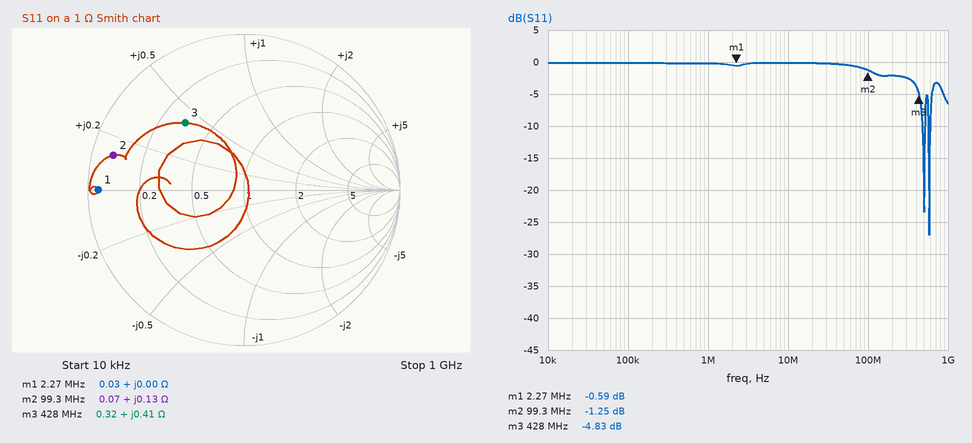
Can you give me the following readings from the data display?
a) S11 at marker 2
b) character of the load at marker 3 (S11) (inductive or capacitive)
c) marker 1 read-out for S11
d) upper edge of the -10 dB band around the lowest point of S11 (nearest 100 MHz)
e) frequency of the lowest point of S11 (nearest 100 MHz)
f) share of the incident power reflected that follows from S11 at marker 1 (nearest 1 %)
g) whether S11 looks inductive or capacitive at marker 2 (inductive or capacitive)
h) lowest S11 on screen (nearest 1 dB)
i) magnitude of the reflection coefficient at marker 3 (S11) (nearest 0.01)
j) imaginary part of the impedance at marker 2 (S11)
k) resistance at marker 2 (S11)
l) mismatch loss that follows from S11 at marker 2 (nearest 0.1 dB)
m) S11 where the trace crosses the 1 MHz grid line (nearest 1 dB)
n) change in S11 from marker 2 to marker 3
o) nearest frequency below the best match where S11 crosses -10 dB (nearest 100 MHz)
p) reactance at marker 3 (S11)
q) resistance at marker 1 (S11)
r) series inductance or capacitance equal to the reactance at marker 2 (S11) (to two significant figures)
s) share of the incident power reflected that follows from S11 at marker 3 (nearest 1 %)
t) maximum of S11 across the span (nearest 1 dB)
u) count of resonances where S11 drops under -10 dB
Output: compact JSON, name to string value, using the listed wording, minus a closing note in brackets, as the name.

{"S11 at marker 2": "-1.25 dB", "character of the load at marker 3 (S11)": "inductive", "marker 1 read-out for S11": "-0.59 dB", "upper edge of the -10 dB band around the lowest point of S11": "600 MHz", "frequency of the lowest point of S11": "600 MHz", "share of the incident power reflected that follows from S11 at marker 1": "87 %", "whether S11 looks inductive or capacitive at marker 2": "inductive", "lowest S11 on screen": "-27 dB", "magnitude of the reflection coefficient at marker 3 (S11)": "0.57", "imaginary part of the impedance at marker 2": "+0.13 Ω", "resistance at marker 2": "0.07 Ω", "mismatch loss that follows from S11 at marker 2": "6.0 dB", "S11 where the trace crosses the 1 MHz grid line": "0 dB", "change in S11 from marker 2 to marker 3": "-3.58 dB", "nearest frequency below the best match where S11 crosses -10 dB": "600 MHz", "reactance at marker 3": "+0.41 Ω", "resistance at marker 1": "0.03 Ω", "series inductance or capacitance equal to the reactance at marker 2 (S11)": "210 pH", "share of the incident power reflected that follows from S11 at marker 3": "33 %", "maximum of S11 across the span": "0 dB", "count of resonances where S11 drops under -10 dB": "2"}
